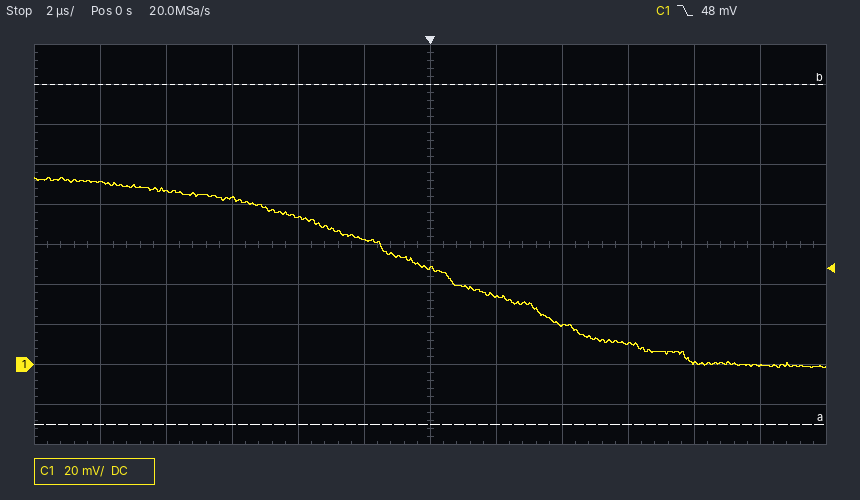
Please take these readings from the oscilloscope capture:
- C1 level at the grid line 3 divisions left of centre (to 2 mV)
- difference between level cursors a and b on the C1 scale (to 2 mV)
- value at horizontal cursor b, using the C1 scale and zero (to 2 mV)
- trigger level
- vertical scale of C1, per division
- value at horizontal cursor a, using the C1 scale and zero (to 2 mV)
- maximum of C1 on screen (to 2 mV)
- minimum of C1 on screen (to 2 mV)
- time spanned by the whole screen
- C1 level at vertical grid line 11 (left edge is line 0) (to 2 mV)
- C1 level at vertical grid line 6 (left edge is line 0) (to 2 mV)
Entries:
84 mV
170 mV
140 mV
48 mV
20 mV
-30 mV
94 mV
-2 mV
24 µs
0 mV
48 mV
